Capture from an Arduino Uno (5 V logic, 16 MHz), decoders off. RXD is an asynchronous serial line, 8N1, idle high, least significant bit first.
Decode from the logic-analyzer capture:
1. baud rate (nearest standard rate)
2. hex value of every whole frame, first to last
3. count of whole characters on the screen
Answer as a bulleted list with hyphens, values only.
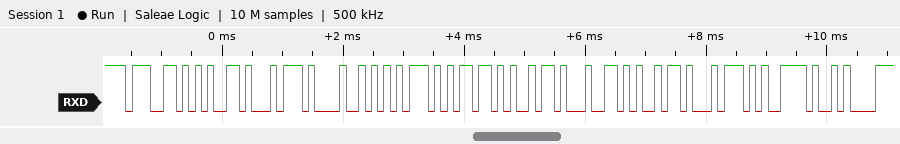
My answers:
- 9600 baud
- 0x67 0x65 0x74 0x48 0x75 0x6D 0x69 0x64 0x69 0x74 0x79 0x0A
- 12
